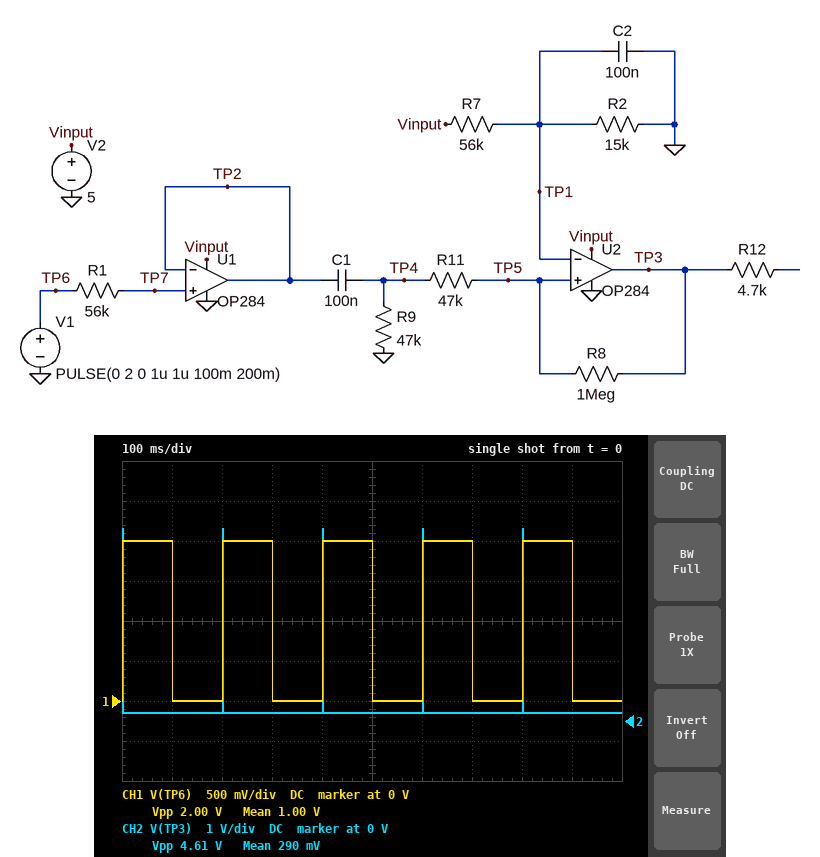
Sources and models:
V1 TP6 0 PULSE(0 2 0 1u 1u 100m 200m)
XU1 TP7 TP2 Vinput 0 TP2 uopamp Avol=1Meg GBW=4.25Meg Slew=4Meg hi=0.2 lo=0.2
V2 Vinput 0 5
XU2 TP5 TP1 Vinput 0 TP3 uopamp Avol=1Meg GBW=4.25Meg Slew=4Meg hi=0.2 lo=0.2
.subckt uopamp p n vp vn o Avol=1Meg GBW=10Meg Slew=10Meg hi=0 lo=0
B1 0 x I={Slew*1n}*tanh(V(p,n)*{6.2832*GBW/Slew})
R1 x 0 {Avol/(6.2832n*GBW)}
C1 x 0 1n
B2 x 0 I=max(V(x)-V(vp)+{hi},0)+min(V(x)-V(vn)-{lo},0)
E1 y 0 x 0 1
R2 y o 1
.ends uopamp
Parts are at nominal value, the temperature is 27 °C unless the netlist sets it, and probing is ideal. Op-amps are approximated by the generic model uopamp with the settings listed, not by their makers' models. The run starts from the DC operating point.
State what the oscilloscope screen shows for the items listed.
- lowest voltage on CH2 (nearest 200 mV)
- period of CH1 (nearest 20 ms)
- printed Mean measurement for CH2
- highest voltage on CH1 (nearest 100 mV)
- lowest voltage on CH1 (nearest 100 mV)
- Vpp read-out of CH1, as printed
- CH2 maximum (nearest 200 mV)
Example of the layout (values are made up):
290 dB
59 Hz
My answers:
200 mV
200 ms
290 mV
2.0 V
0 V
2.00 V
4.8 V
